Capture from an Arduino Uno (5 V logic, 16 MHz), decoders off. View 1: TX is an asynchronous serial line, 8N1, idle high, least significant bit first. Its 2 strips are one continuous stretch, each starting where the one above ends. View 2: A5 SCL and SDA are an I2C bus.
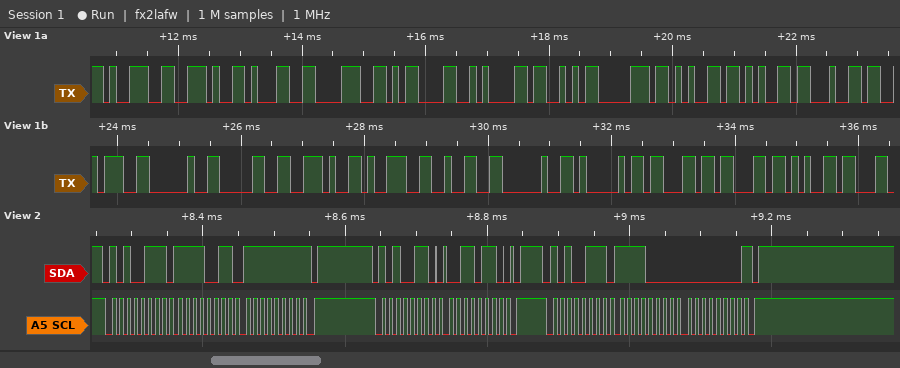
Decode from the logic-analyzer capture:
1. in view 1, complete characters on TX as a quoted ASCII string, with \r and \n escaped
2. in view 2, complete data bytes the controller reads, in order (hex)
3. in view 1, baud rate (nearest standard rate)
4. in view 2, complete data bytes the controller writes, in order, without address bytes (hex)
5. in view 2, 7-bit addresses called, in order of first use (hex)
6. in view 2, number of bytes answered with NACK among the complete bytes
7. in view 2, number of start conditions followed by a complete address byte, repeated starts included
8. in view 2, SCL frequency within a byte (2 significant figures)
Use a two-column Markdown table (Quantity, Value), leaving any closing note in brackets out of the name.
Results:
| Quantity | Value |
|---|---|
| in view 1, complete characters on TX as a quoted ASCII string, with \r and \n escaped | "9.18\r\nSpeed: 0.92 Acce" |
| in view 2, complete data bytes the controller reads, in order | F3 FF F0 00 |
| in view 1, baud rate | 9600 baud |
| in view 2, complete data bytes the controller writes, in order, without address bytes | 36 |
| in view 2, 7-bit addresses called, in order of first use | 0x53 |
| in view 2, number of bytes answered with NACK among the complete bytes | 2 |
| in view 2, number of start conditions followed by a complete address byte, repeated starts included | 3 |
| in view 2, SCL frequency within a byte | 100 kHz |
